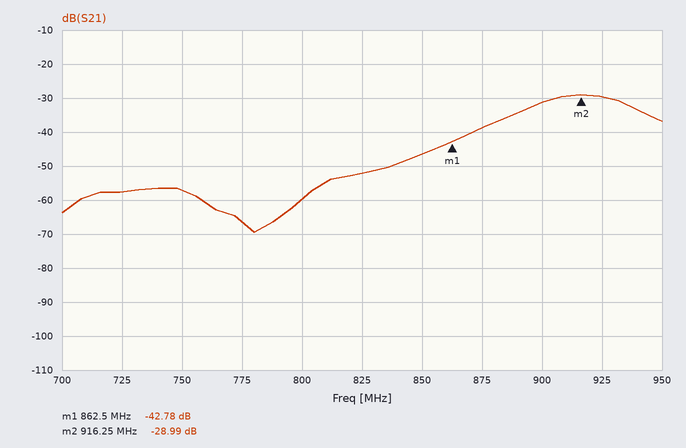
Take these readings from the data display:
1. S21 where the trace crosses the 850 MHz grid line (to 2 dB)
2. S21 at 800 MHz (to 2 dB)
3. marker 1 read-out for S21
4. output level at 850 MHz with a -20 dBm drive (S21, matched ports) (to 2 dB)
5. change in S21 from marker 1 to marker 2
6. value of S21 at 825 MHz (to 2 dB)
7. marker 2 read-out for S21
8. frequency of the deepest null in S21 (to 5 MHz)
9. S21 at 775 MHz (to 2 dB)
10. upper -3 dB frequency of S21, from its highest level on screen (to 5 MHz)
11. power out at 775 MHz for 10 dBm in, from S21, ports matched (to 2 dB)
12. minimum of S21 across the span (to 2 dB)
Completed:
-46 dB
-60 dB
-42.78 dB
-66 dBm
13.79 dB
-52 dB
-28.99 dB
780 MHz
-66 dB
935 MHz
-56 dBm
-70 dB
